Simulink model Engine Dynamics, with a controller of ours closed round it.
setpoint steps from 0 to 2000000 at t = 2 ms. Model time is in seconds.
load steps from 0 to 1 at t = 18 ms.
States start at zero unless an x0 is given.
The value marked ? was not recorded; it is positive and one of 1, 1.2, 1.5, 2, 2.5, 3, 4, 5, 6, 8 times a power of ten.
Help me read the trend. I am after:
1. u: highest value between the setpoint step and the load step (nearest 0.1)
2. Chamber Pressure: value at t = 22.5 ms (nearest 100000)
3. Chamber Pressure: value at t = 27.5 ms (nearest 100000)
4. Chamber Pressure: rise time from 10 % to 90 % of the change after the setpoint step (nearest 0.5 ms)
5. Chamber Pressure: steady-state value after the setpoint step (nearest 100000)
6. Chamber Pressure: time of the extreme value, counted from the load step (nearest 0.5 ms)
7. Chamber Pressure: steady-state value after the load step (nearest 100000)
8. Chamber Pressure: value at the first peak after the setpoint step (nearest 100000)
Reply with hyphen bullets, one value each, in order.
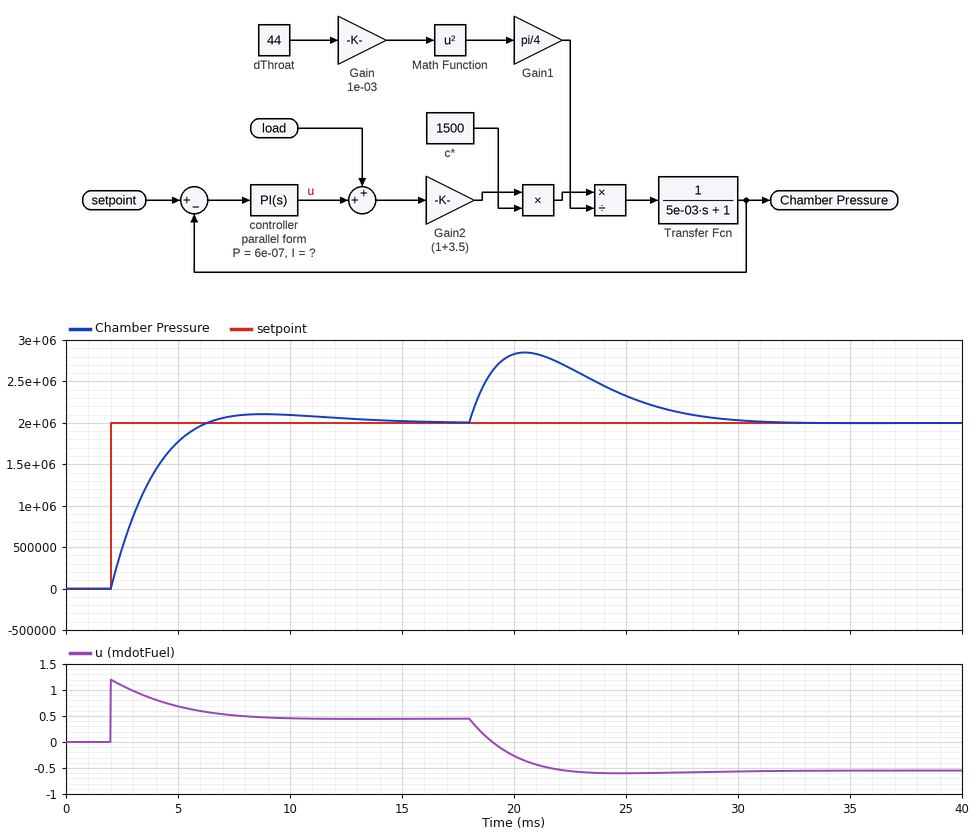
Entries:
- 1.2
- 2700000
- 2100000
- 3.0 ms
- 2000000
- 2.5 ms
- 2000000
- 2100000
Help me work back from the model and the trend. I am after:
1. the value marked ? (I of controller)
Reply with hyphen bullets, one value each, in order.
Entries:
- 0.0002
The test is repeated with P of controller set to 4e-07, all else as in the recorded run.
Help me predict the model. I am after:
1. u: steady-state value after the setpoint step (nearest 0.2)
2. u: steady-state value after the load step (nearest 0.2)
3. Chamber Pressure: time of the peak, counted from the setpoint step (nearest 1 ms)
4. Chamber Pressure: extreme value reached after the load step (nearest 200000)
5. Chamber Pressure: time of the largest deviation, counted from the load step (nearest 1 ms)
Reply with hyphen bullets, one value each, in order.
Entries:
- 0.4
- -0.6
- 7 ms
- 3000000
- 3 ms
